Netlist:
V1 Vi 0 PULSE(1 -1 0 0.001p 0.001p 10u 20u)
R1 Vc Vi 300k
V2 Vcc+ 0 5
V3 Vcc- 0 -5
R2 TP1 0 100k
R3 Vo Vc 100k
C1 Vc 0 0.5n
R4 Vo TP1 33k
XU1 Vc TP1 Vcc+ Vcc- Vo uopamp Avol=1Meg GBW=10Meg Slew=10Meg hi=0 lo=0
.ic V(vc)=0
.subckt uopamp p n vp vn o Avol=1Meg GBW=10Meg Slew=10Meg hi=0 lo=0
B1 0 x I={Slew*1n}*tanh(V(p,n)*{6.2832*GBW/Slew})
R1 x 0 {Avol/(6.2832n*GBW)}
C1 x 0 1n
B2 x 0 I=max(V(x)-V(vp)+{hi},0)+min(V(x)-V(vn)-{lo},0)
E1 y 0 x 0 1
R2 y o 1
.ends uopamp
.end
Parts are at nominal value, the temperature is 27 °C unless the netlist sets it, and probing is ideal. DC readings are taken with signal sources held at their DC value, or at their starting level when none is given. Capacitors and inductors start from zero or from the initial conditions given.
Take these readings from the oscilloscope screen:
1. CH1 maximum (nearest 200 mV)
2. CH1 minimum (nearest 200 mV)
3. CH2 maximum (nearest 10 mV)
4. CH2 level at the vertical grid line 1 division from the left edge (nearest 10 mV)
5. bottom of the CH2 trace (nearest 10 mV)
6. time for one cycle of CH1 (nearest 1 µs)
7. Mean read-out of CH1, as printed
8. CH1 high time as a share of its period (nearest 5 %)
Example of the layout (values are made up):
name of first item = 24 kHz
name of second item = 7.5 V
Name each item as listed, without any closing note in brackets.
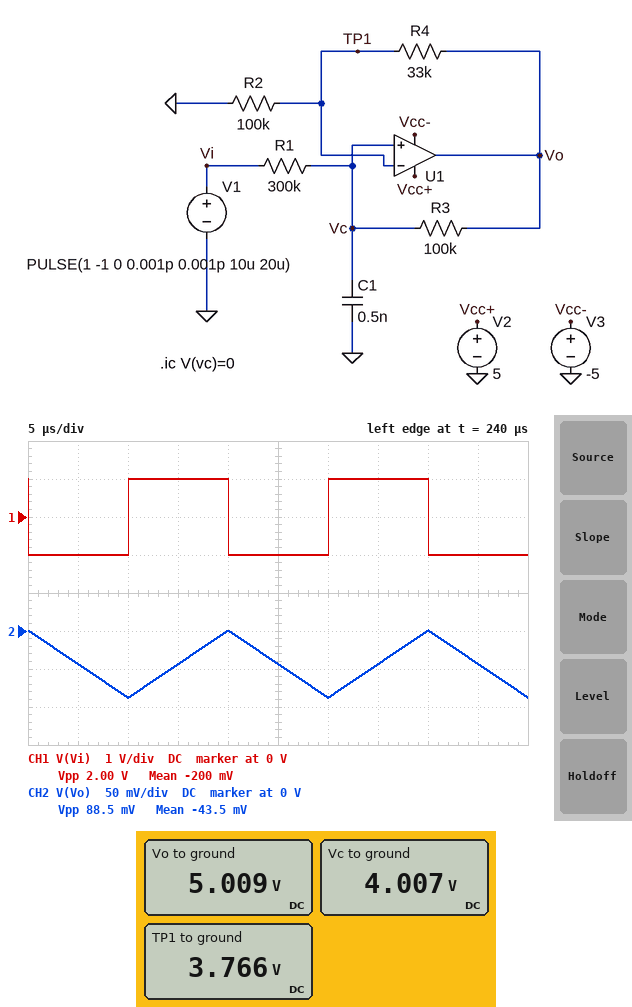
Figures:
CH1 maximum = 1.0 V
CH1 minimum = -1.0 V
CH2 maximum = 0 V
CH2 level at the vertical grid line 1 division from the left edge = -40 mV
bottom of the CH2 trace = -90 mV
time for one cycle of CH1 = 20 µs
Mean read-out of CH1, as printed = -200 mV
CH1 high time as a share of its period = 50 %
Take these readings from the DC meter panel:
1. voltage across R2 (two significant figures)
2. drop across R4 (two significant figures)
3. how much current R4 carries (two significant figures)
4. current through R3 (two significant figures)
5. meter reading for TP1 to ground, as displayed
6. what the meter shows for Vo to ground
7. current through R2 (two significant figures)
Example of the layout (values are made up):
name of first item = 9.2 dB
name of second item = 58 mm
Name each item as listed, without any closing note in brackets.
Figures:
voltage across R2 = 3.8 V
drop across R4 = 1.2 V
how much current R4 carries = 38 µA
current through R3 = 10 µA
meter reading for TP1 to ground, as displayed = 3.766 V
what the meter shows for Vo to ground = 5.009 V
current through R2 = 38 µA
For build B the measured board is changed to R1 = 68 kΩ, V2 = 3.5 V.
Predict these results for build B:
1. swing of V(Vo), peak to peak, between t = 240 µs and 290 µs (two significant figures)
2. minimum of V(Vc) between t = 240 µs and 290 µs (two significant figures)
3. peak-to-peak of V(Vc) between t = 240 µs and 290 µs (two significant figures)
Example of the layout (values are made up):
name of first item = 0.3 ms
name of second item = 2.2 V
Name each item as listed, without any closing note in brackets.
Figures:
swing of V(Vo), peak to peak, between t = 240 µs and 290 µs = 390 mV
minimum of V(Vc) between t = 240 µs and 290 µs = -150 mV
peak-to-peak of V(Vc) between t = 240 µs and 290 µs = 290 mV
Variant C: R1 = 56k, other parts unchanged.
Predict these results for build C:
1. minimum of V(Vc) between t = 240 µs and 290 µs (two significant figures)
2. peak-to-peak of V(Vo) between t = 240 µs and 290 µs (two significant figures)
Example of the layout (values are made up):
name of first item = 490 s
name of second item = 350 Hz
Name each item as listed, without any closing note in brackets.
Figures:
minimum of V(Vc) between t = 240 µs and 290 µs = -180 mV
peak-to-peak of V(Vo) between t = 240 µs and 290 µs = 470 mV
